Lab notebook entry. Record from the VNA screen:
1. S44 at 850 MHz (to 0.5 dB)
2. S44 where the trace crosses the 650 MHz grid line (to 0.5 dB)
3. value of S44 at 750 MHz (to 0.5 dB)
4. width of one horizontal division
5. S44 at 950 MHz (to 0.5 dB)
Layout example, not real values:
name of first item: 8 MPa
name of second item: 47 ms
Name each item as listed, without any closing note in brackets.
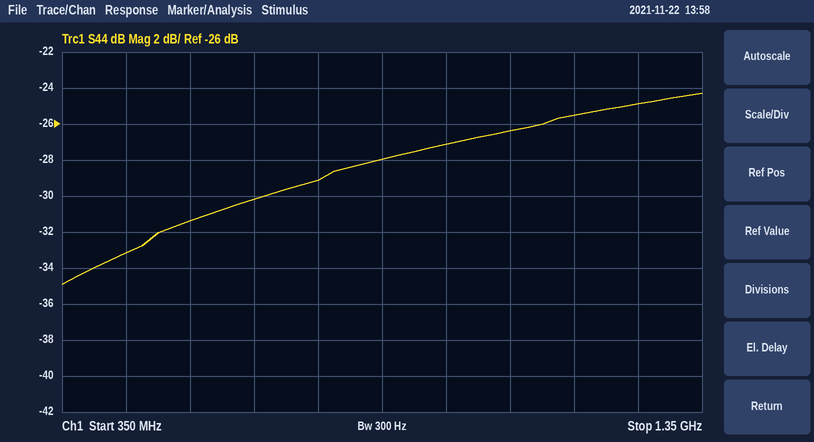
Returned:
S44 at 850 MHz: -28.0 dB
S44 where the trace crosses the 650 MHz grid line: -30.0 dB
value of S44 at 750 MHz: -29.0 dB
width of one horizontal division: 100 MHz
S44 at 950 MHz: -27.0 dB
